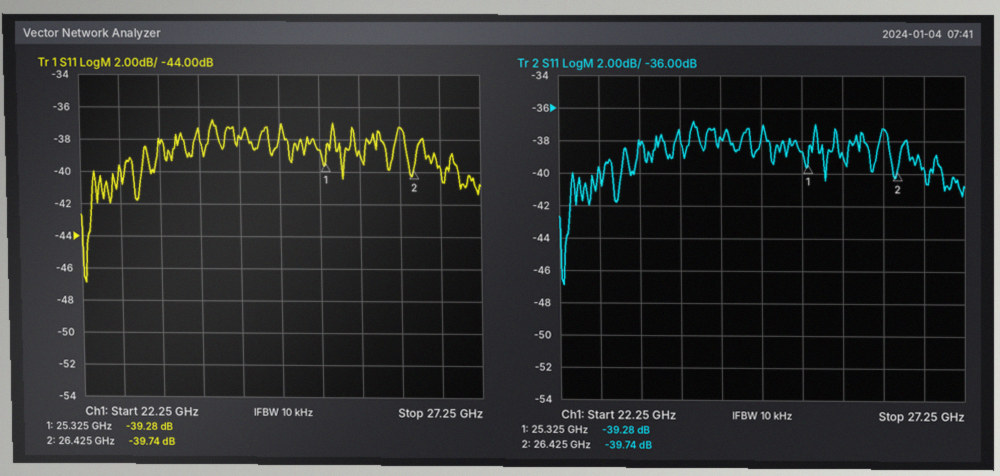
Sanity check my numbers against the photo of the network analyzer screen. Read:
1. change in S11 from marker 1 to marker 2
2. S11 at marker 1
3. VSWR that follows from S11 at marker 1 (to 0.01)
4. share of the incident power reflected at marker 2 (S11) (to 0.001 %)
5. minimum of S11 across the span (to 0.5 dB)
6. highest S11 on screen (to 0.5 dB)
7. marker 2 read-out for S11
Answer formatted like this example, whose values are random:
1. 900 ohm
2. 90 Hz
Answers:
1. -0.46 dB
2. -39.28 dB
3. 1.02
4. 0.011 %
5. -47.0 dB
6. -37.0 dB
7. -39.74 dB
